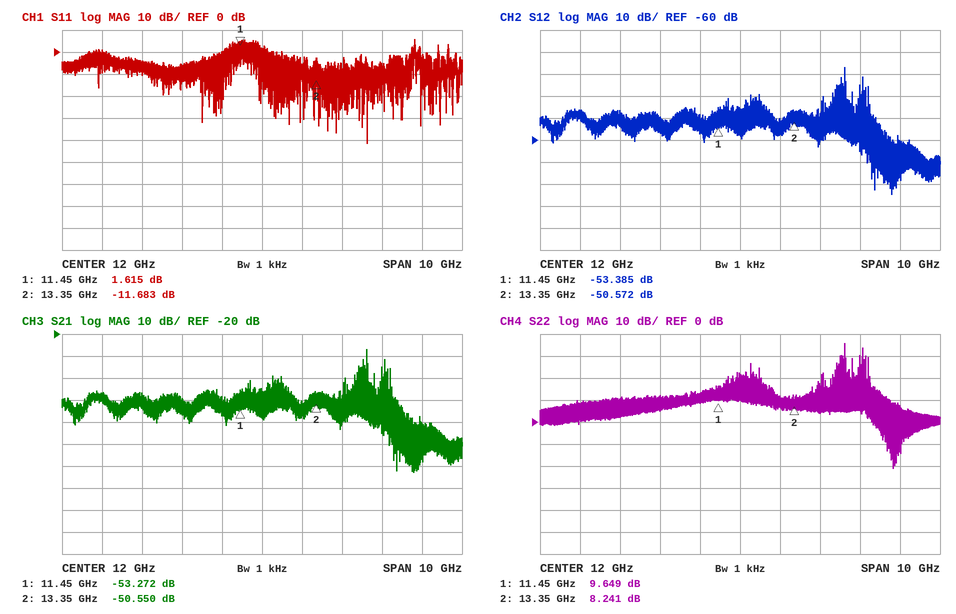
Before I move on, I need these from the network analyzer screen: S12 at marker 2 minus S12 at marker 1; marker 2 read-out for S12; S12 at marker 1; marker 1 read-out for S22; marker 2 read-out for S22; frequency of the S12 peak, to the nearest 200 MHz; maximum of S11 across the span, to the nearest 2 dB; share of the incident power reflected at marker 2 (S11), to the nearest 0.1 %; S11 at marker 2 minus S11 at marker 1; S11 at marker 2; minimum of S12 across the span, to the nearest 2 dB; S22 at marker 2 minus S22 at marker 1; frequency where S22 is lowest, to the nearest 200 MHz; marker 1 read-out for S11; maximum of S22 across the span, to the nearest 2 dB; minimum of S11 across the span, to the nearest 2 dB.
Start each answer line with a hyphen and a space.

- 2.813 dB
- -50.572 dB
- -53.385 dB
- 9.649 dB
- 8.241 dB
- 14.6 GHz
- 6 dB
- 6.8 %
- -13.298 dB
- -11.683 dB
- -84 dB
- -1.408 dB
- 15.8 GHz
- 1.615 dB
- 36 dB
- -42 dB
